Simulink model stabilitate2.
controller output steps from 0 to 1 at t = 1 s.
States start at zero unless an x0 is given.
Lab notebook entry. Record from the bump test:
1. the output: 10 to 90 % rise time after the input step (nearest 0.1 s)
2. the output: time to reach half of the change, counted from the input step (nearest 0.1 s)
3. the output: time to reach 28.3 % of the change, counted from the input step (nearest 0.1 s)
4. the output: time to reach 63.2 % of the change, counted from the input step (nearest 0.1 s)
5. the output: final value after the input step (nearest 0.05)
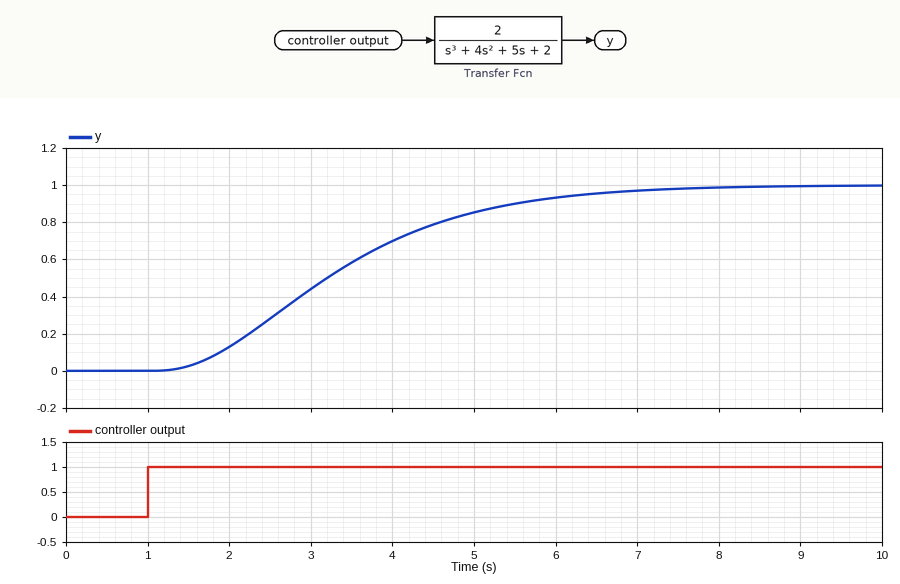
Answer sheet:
3.6 s
2.2 s
1.5 s
2.7 s
1.00
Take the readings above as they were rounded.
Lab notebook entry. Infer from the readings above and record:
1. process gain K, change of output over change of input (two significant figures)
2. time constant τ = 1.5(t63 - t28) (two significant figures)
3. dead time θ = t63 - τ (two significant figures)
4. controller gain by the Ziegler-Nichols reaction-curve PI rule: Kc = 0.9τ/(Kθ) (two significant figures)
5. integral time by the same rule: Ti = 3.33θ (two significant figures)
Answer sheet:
1.0
1.8 s
0.90 s
1.8
3.0 s
